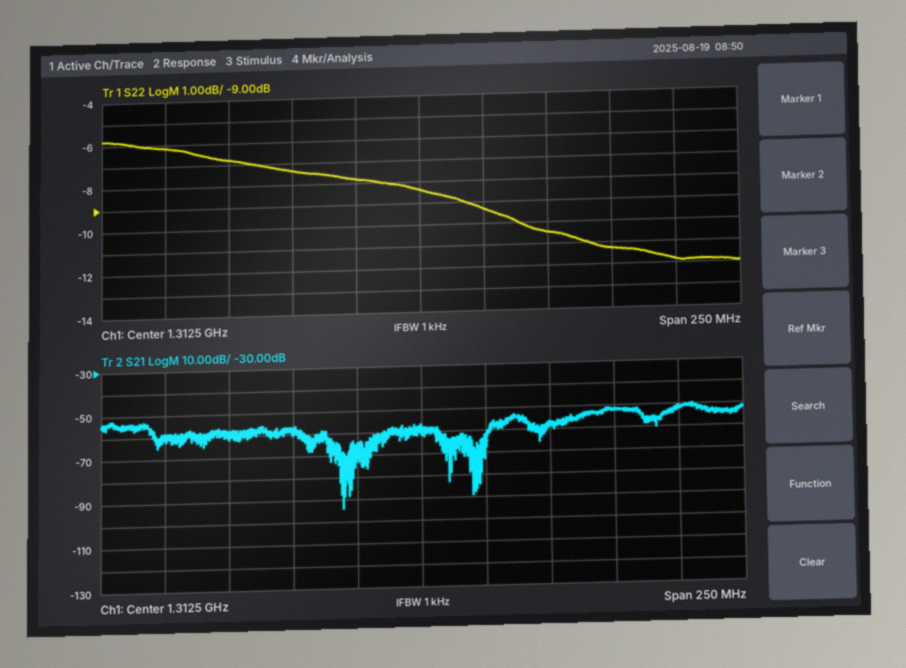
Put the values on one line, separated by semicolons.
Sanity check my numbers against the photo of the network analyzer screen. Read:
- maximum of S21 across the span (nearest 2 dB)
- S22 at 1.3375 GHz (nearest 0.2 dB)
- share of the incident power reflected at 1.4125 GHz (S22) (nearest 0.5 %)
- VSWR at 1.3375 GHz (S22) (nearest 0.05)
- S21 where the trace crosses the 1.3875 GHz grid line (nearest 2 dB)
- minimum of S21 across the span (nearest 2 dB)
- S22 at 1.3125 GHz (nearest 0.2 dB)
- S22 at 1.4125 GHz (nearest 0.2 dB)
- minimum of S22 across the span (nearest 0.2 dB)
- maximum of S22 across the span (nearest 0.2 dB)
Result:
-50 dB; -9.4 dB; 6.5 %; 2.05; -52 dB; -94 dB; -8.4 dB; -11.8 dB; -12.0 dB; -5.8 dB
